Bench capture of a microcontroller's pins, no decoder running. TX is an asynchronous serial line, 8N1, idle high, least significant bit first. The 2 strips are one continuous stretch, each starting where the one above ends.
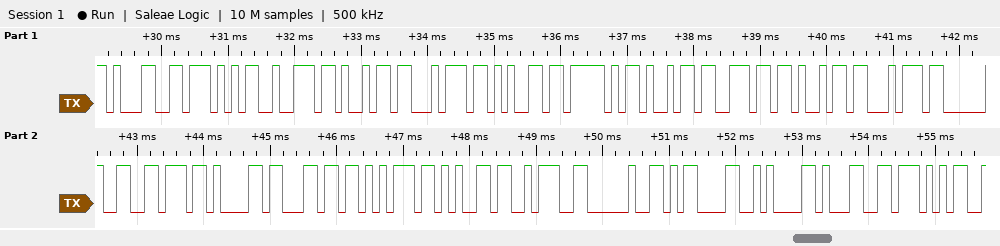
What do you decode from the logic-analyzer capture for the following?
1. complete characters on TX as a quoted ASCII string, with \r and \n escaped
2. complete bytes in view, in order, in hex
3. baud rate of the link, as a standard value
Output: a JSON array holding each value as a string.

["\"1Write_init value: \\r\\n1W\"", "31 57 72 69 74 65 5F 69 6E 69 74 20 76 61 6C 75 65 3A 20 0D 0A 31 57", "9600 baud"]
